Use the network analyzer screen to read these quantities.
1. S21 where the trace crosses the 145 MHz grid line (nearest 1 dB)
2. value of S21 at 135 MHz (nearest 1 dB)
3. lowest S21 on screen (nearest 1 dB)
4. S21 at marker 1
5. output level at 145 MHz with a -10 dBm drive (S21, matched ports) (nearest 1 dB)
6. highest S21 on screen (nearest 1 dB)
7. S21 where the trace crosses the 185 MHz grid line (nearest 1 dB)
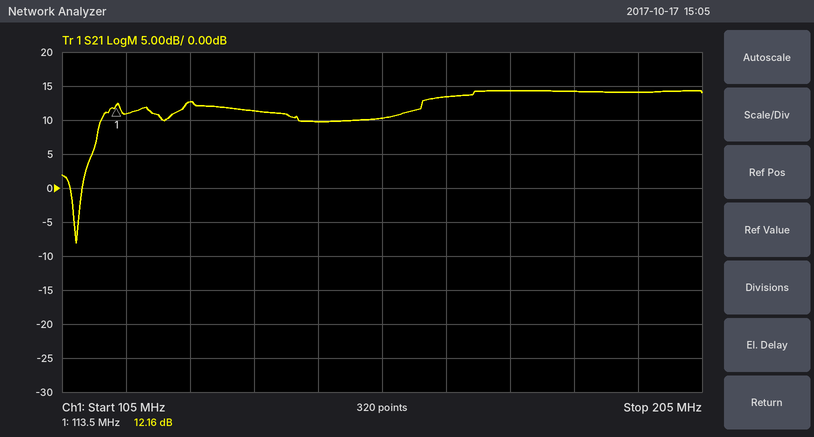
10 dB
11 dB
-8 dB
12.16 dB
0 dBm
14 dB
14 dB
